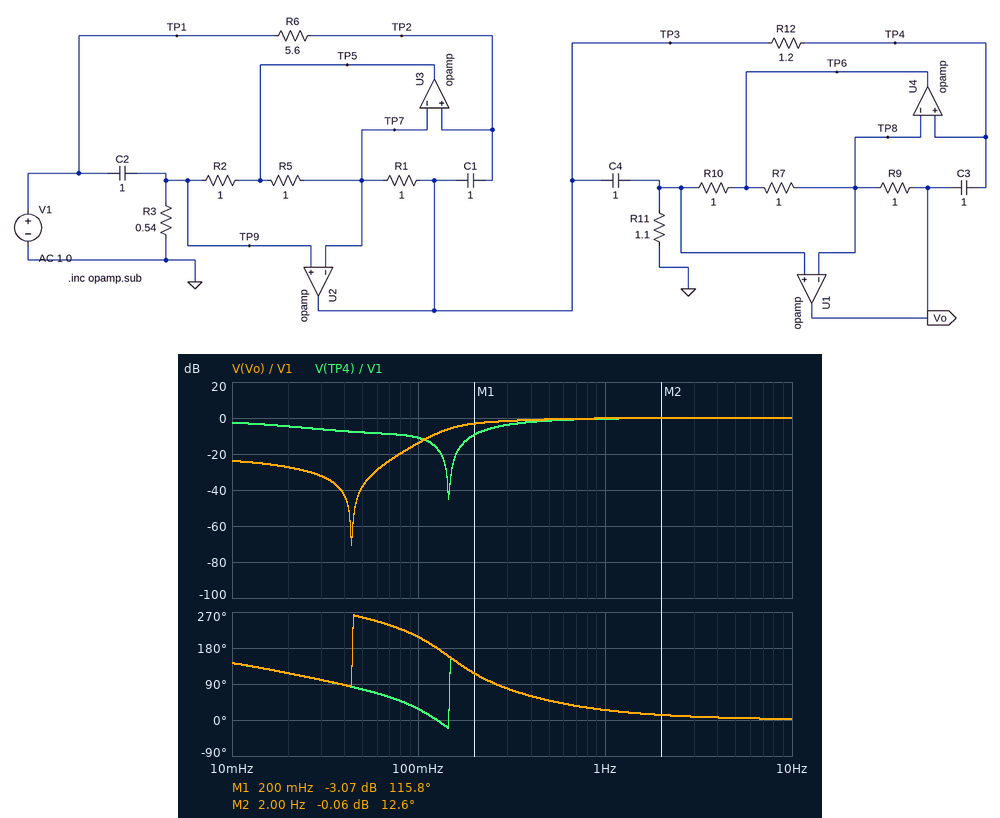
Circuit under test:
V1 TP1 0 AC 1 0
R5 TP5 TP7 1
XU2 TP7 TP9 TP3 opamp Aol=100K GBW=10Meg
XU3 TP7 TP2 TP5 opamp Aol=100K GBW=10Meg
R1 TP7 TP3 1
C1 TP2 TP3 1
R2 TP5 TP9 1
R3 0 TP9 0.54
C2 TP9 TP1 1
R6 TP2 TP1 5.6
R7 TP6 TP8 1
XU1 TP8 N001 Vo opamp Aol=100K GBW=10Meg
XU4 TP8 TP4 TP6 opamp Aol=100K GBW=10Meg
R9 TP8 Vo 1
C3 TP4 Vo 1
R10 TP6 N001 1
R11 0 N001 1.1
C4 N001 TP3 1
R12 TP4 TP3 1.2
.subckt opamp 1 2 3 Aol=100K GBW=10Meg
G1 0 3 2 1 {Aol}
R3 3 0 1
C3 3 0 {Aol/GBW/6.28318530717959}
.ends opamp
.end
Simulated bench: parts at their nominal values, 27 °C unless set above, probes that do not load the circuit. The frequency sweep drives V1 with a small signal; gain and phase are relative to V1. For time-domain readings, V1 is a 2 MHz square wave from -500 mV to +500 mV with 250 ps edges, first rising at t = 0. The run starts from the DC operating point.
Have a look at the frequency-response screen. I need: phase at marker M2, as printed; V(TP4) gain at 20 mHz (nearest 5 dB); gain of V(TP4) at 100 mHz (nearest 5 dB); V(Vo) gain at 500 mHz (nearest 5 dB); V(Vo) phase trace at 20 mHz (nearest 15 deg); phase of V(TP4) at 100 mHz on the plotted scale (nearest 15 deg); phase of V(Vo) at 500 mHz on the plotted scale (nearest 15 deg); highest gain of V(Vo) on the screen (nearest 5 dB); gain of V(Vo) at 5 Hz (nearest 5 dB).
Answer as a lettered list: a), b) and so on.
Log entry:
a) 12.6 deg
b) -5 dB
c) -10 dB
d) 0 dB
e) 120 deg
f) 30 deg
g) 45 deg
h) 0 dB
i) 0 dB
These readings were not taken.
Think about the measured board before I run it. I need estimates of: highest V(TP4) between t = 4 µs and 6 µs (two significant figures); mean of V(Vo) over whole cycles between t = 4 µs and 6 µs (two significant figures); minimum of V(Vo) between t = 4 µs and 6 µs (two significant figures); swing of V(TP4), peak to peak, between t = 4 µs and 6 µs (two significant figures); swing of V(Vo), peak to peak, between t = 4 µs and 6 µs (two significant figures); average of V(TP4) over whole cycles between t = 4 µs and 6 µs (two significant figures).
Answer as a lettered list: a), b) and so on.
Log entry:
a) 1.8 V
b) 540 mV
c) -380 mV
d) 1.8 V
e) 1.8 V
f) 930 mV
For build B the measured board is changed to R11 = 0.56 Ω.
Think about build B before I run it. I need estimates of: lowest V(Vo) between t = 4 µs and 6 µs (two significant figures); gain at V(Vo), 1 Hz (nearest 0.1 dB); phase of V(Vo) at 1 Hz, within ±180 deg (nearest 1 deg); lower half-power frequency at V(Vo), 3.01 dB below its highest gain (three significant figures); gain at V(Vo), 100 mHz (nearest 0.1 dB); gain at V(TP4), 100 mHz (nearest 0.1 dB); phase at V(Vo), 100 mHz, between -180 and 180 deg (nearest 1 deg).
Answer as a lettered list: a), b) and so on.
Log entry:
a) -750 mV
b) -0.3 dB
c) 33 deg
d) 270 mHz
e) -7.9 dB
f) -15.5 dB
g) -169 deg
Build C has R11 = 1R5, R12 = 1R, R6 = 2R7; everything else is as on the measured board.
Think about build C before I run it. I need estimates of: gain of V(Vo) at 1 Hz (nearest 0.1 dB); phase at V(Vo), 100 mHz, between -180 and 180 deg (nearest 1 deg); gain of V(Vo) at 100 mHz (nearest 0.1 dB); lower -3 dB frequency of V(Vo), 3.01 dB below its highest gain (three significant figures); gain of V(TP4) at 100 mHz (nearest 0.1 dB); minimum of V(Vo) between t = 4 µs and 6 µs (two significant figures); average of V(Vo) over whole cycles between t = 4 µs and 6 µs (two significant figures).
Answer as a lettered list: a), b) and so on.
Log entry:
a) -0.1 dB
b) -126 deg
c) -25.9 dB
d) 163 mHz
e) -6.0 dB
f) -270 mV
g) 640 mV
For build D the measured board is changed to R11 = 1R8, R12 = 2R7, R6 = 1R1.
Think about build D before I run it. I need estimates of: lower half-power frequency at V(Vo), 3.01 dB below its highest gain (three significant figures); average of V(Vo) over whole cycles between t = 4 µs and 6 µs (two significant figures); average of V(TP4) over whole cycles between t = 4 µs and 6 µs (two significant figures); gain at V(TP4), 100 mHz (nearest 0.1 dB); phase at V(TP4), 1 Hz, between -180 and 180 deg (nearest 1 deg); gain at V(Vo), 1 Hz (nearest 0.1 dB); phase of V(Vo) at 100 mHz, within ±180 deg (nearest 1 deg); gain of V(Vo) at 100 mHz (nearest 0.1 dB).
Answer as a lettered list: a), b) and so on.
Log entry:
a) 108 mHz
b) 690 mV
c) 930 mV
d) -23.9 dB
e) 22 deg
f) 0 dB
g) -160 deg
h) -4.4 dB
